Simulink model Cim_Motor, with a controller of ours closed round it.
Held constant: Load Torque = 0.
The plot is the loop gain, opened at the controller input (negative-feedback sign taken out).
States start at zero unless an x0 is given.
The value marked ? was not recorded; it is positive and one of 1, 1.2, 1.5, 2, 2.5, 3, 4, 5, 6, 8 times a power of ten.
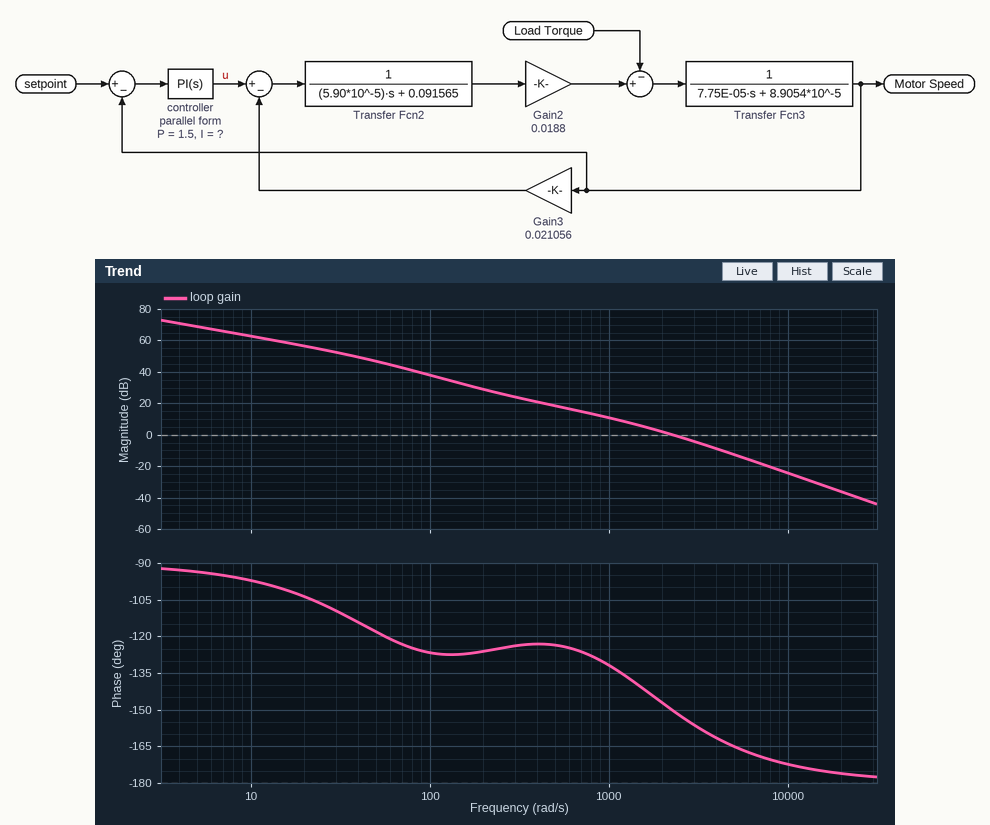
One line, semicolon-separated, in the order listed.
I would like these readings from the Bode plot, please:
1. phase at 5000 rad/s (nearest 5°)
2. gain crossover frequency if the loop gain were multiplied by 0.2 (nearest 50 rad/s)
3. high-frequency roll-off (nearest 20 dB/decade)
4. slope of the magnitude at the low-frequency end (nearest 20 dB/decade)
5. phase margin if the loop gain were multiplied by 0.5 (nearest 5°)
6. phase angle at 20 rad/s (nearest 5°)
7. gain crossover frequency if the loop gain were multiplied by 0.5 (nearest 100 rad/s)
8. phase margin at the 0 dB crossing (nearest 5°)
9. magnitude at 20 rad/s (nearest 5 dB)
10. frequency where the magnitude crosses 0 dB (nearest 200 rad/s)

-165°; 750 rad/s; -40 dB/decade; -20 dB/decade; 40°; -105°; 1500 rad/s; 30°; 55 dB; 2200 rad/s
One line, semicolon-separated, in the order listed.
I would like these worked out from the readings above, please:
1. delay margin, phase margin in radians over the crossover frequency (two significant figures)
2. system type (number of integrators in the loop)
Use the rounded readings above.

0.00024 s; 1
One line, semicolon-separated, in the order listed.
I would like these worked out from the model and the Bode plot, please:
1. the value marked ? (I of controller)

300
